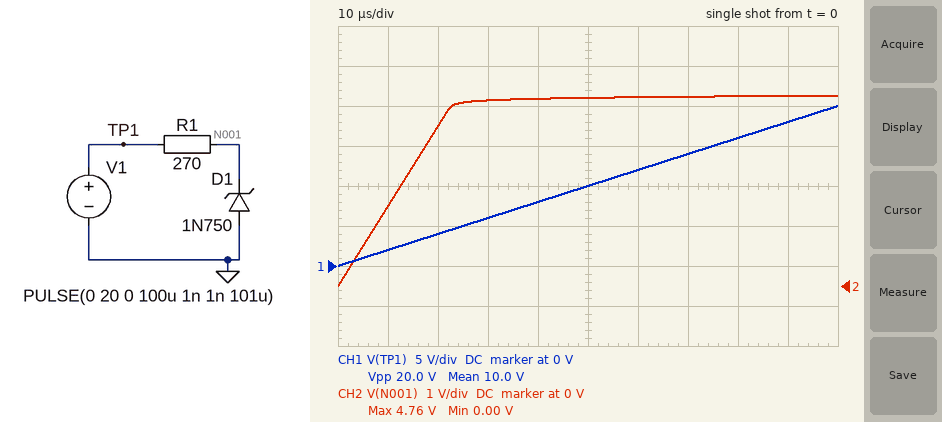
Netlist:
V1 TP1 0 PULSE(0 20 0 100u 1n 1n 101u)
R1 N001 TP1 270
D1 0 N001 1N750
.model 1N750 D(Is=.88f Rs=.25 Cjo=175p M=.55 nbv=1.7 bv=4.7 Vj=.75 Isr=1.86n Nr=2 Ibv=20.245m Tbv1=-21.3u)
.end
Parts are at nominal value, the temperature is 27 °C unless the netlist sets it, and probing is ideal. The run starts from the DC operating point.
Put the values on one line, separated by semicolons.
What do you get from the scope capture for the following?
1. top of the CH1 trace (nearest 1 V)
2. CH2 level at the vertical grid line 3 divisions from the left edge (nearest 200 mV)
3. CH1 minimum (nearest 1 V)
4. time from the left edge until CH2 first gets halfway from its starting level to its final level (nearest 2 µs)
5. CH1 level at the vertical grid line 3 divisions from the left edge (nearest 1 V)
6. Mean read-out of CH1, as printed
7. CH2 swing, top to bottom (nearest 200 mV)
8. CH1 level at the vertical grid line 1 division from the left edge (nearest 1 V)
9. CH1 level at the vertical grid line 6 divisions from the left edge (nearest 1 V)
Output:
20 V; 4.6 V; 0 V; 12 µs; 6 V; 10.0 V; 4.8 V; 2 V; 12 V
